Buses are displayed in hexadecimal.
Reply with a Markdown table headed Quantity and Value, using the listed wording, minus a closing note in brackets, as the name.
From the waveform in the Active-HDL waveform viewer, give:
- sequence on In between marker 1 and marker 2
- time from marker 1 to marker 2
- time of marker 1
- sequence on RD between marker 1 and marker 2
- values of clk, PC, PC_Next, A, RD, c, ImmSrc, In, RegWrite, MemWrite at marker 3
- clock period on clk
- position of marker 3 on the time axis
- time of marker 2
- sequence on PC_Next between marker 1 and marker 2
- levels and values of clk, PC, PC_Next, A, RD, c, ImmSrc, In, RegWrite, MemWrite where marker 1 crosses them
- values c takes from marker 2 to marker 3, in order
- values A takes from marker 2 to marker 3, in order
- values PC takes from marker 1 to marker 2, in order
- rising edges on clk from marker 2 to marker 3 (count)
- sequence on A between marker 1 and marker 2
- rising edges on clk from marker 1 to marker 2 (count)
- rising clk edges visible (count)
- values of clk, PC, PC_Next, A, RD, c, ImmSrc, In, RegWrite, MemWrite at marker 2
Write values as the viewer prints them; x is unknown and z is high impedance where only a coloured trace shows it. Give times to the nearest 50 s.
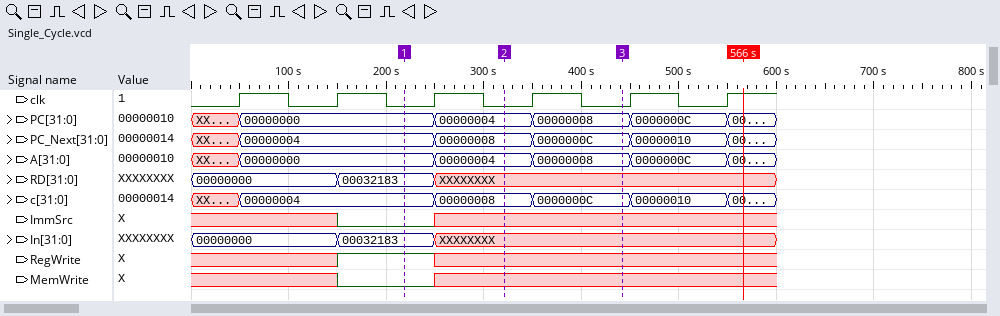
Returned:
| Quantity | Value |
|---|---|
| sequence on In between marker 1 and marker 2 | 00032183, XXXXXXXX |
| time from marker 1 to marker 2 | 100 s |
| time of marker 1 | 200 s |
| sequence on RD between marker 1 and marker 2 | 00032183, XXXXXXXX |
| values of clk, PC, PC_Next, A, RD, c, ImmSrc, In, RegWrite, MemWrite at marker 3 | clk=0, PC=00000008, PC_Next=0000000C, A=00000008, RD=XXXXXXXX, c=0000000C, ImmSrc=x, In=XXXXXXXX, RegWrite=x, MemWrite=x |
| clock period on clk | 100 s |
| position of marker 3 on the time axis | 450 s |
| time of marker 2 | 300 s |
| sequence on PC_Next between marker 1 and marker 2 | 00000004, 00000008 |
| levels and values of clk, PC, PC_Next, A, RD, c, ImmSrc, In, RegWrite, MemWrite where marker 1 crosses them | clk=0, PC=00000000, PC_Next=00000004, A=00000000, RD=00032183, c=00000004, ImmSrc=0, In=00032183, RegWrite=1, MemWrite=0 |
| values c takes from marker 2 to marker 3, in order | 00000008, 0000000C |
| values A takes from marker 2 to marker 3, in order | 00000004, 00000008 |
| values PC takes from marker 1 to marker 2, in order | 00000000, 00000004 |
| rising edges on clk from marker 2 to marker 3 | 1 |
| sequence on A between marker 1 and marker 2 | 00000000, 00000004 |
| rising edges on clk from marker 1 to marker 2 | 1 |
| rising clk edges visible | 6 |
| values of clk, PC, PC_Next, A, RD, c, ImmSrc, In, RegWrite, MemWrite at marker 2 | clk=0, PC=00000004, PC_Next=00000008, A=00000004, RD=XXXXXXXX, c=00000008, ImmSrc=x, In=XXXXXXXX, RegWrite=x, MemWrite=x |
